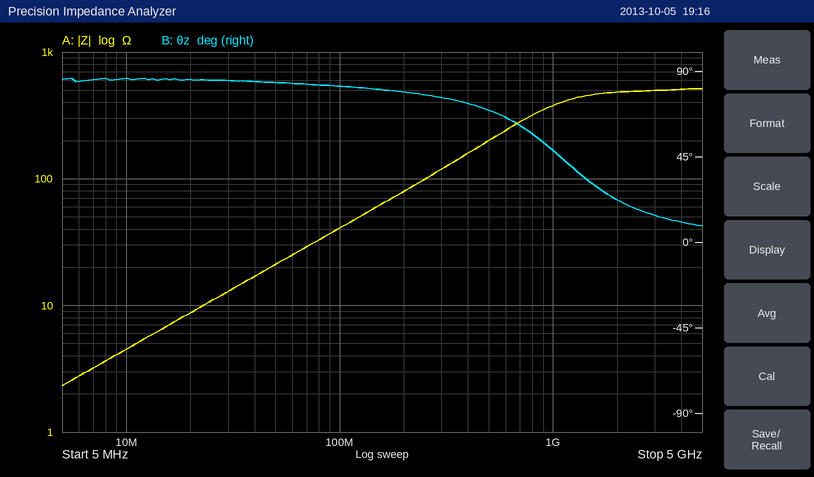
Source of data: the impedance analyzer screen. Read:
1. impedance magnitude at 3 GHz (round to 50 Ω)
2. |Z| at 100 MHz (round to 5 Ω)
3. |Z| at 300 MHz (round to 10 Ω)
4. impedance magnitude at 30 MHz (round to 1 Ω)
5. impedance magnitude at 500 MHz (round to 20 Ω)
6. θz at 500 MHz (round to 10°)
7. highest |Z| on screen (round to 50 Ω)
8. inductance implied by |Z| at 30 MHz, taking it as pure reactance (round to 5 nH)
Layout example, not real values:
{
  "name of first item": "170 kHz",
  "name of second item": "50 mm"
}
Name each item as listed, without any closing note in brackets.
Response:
{
  "impedance magnitude at 3 GHz": "500 Ω",
  "|Z| at 100 MHz": "40 Ω",
  "|Z| at 300 MHz": "120 Ω",
  "impedance magnitude at 30 MHz": "13 Ω",
  "impedance magnitude at 500 MHz": "200 Ω",
  "θz at 500 MHz": "70°",
  "highest |Z| on screen": "500 Ω",
  "inductance implied by |Z| at 30 MHz, taking it as pure reactance": "70 nH"
}
